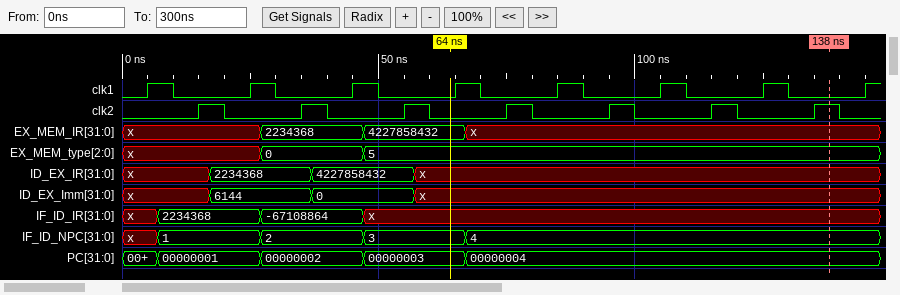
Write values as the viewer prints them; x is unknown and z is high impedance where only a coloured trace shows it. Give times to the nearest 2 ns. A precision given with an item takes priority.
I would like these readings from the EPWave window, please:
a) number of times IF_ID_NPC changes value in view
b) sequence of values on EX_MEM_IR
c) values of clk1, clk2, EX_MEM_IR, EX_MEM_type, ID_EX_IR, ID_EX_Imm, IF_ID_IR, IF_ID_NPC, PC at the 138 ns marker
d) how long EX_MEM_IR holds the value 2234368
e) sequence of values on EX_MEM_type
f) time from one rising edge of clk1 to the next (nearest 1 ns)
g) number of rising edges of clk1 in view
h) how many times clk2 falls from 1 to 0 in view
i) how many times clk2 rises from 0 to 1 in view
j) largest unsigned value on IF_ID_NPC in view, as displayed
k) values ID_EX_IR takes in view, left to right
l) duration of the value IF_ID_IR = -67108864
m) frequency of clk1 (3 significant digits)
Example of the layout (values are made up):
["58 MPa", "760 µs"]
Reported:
["4", "x, 2234368, 4227858432, x", "clk1=0, clk2=1, EX_MEM_IR=x, EX_MEM_type=5, ID_EX_IR=x, ID_EX_Imm=x, IF_ID_IR=x, IF_ID_NPC=4, PC=00000004", "20 ns", "x, 0, 5", "20 ns", "8", "7", "7", "4", "x, 2234368, 4227858432, x", "20 ns", "50.0 MHz"]
